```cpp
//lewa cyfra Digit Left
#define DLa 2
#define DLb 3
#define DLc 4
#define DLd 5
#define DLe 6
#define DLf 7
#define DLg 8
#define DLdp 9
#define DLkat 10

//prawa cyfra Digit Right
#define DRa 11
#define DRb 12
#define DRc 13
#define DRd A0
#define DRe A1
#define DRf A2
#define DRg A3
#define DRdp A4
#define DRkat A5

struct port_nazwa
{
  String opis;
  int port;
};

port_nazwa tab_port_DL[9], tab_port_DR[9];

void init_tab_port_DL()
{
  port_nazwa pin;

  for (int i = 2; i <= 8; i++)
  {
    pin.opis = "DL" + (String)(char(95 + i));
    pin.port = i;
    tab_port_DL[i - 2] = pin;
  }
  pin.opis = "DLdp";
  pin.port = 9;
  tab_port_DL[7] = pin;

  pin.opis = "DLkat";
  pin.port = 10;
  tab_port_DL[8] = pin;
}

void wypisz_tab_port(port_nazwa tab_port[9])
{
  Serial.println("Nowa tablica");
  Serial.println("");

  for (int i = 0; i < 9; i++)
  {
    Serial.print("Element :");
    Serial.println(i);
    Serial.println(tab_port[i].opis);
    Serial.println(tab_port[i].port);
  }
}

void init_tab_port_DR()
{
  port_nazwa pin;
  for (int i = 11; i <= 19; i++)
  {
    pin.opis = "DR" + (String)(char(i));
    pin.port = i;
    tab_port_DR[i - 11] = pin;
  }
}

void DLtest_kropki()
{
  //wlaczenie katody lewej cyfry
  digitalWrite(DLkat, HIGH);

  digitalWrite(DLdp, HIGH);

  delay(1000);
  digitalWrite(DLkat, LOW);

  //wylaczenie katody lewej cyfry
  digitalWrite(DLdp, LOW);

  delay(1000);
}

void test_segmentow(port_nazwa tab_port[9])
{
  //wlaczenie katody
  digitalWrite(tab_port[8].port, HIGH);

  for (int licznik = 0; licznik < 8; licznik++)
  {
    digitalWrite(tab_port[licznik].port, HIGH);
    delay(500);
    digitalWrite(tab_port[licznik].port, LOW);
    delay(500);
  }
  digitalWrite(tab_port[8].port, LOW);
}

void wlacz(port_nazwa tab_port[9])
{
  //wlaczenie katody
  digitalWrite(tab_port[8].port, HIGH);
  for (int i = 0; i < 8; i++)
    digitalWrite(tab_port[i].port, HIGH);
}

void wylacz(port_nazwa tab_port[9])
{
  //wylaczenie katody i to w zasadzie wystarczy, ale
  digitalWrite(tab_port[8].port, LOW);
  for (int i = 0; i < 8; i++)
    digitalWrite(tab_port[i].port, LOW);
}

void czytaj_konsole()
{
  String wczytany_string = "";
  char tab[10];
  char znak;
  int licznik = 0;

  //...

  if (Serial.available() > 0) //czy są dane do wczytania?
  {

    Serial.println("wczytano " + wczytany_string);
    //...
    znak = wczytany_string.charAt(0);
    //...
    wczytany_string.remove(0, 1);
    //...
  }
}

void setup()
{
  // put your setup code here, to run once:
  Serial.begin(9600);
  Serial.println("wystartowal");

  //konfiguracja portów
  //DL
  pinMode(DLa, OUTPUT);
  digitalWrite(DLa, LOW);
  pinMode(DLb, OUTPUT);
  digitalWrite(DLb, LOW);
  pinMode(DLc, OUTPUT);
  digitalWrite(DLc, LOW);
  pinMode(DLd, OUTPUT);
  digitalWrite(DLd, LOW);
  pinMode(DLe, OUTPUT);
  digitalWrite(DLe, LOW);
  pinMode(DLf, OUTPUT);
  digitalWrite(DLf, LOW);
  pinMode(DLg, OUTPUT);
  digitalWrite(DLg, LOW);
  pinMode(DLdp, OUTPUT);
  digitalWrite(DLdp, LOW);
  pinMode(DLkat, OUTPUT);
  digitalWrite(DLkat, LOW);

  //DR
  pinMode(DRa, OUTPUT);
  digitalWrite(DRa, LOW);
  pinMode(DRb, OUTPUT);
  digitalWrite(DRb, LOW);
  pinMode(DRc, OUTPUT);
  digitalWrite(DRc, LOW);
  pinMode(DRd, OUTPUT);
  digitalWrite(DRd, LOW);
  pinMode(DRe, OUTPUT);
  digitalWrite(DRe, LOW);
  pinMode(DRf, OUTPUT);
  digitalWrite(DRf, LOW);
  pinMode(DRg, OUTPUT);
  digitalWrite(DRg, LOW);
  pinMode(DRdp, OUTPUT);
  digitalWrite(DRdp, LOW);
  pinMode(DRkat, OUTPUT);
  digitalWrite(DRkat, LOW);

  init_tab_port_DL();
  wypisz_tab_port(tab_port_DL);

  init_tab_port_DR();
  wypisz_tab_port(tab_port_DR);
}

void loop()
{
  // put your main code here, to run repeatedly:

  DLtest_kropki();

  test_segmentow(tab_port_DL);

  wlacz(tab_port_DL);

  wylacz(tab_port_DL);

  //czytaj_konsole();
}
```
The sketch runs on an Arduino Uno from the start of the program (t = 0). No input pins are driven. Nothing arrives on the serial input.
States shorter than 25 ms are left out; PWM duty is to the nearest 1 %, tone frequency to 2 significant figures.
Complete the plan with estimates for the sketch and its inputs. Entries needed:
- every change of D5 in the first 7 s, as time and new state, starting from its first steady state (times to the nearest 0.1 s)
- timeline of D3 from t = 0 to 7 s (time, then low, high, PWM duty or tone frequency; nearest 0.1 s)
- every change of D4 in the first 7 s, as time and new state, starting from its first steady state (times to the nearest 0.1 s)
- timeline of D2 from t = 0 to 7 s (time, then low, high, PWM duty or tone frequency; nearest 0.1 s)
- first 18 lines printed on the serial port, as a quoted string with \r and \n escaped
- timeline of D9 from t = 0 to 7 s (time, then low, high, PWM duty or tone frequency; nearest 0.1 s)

0 s low; 5.4 s high; 5.9 s low
0 s low; 3.4 s high; 3.9 s low
0 s low; 4.4 s high; 4.9 s low
0 s low; 2.4 s high; 2.9 s low
"wystartowal\r\nNowa tablica\r\n\r\nElement :0\r\nDLa\r\n2\r\nElement :1\r\nDLb\r\n3\r\nElement :2\r\nDLc\r\n4\r\nElement :3\r\nDLd\r\n5\r\nElement :4\r\nDLe\r\n6\r\n"
0 s low; 0.4 s high; 1.4 s low
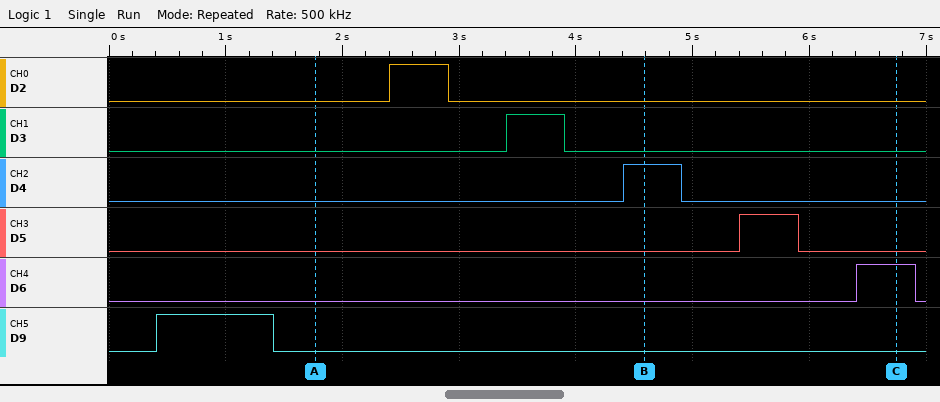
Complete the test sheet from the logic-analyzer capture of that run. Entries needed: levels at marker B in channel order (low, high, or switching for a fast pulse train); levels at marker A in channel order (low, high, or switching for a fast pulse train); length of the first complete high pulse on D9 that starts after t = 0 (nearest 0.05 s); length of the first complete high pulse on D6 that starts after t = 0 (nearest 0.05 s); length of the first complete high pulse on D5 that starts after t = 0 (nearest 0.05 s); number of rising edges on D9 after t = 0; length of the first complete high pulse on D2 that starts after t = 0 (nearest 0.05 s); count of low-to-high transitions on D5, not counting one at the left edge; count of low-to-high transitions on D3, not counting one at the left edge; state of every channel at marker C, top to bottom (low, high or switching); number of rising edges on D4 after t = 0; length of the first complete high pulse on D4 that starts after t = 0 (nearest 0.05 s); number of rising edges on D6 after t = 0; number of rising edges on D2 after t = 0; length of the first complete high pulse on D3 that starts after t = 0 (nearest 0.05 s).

D2 low, D3 low, D4 high, D5 low, D6 low, D9 low
D2 low, D3 low, D4 low, D5 low, D6 low, D9 low
1.00 s
0.50 s
0.50 s
1
0.50 s
1
1
D2 low, D3 low, D4 low, D5 low, D6 high, D9 low
1
0.50 s
1
1
0.50 s
